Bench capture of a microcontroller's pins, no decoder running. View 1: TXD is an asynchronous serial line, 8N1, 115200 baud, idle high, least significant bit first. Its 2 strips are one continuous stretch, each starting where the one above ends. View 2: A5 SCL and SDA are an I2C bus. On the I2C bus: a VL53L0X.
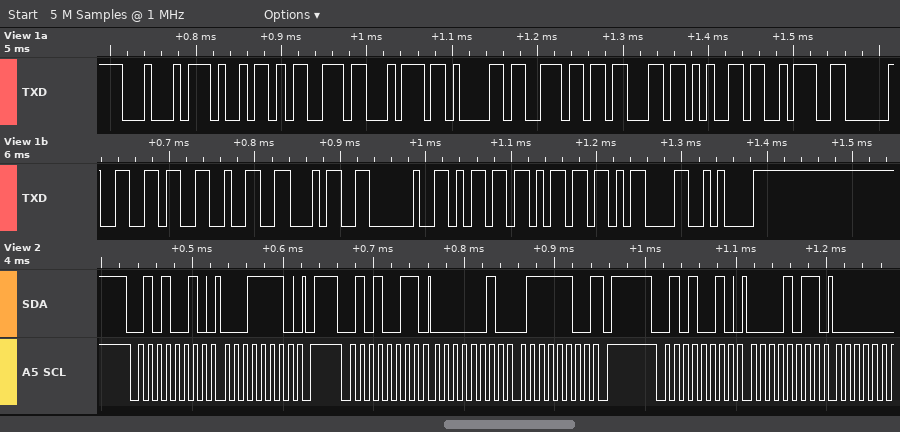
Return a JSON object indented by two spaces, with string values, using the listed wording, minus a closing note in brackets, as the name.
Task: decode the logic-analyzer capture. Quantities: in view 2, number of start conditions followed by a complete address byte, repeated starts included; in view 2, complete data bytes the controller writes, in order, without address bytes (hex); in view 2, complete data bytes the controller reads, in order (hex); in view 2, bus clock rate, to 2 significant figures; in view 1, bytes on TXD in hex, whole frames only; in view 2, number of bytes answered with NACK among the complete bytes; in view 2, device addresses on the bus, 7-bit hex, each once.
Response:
{
  "in view 2, number of start conditions followed by a complete address byte, repeated starts included": "3",
  "in view 2, complete data bytes the controller writes, in order, without address bytes": "1E 0B",
  "in view 2, complete data bytes the controller reads, in order": "02 7C",
  "in view 2, bus clock rate, to 2 significant figures": "100 kHz",
  "in view 1, bytes on TXD in hex, whole frames only": "44 69 73 74 61 6E 63 65 3A 20 36 32 34 20 6D 6D 0D 0A",
  "in view 2, number of bytes answered with NACK among the complete bytes": "1",
  "in view 2, device addresses on the bus, 7-bit hex, each once": "0x29"
}
